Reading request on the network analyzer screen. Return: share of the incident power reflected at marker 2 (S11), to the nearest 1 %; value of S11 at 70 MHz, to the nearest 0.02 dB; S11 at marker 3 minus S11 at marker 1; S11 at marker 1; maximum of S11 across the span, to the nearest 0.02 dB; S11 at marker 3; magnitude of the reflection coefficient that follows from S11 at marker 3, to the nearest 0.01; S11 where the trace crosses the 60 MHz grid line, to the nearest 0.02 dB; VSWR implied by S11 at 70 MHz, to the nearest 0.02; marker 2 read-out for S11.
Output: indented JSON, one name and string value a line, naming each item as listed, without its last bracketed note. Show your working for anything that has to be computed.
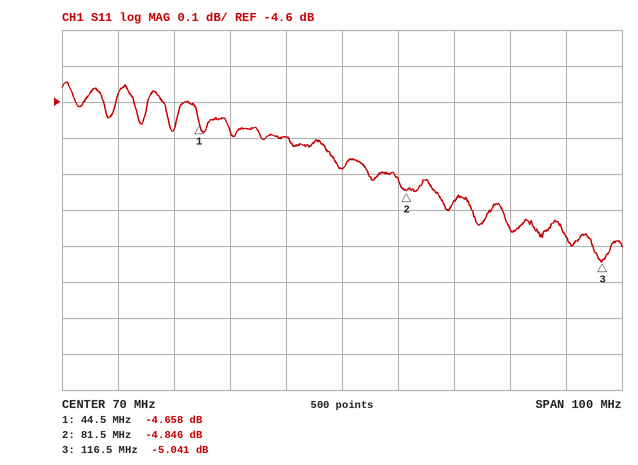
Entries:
{
  "share of the incident power reflected at marker 2 (S11), to the nearest 1 %": "10^(-4.846/10) ≈ 33 %",
  "value of S11 at 70 MHz, to the nearest 0.02 dB": "-4.78 dB",
  "S11 at marker 3 minus S11 at marker 1": "-5.041 − (-4.658) = -0.383 dB",
  "S11 at marker 1": "-4.658 dB",
  "maximum of S11 across the span, to the nearest 0.02 dB": "-4.54 dB",
  "S11 at marker 3": "-5.041 dB",
  "magnitude of the reflection coefficient that follows from S11 at marker 3, to the nearest 0.01": "10^(-5.041/20) ≈ 0.56",
  "S11 where the trace crosses the 60 MHz grid line, to the nearest 0.02 dB": "-4.70 dB",
  "VSWR implied by S11 at 70 MHz, to the nearest 0.02": "|Γ| = 10^(-4.78/20) = 0.5768; VSWR = (1 + 0.5768)/(1 − 0.5768) ≈ 3.73, so 3.72 to the nearest 0.02",
  "marker 2 read-out for S11": "-4.846 dB"
}
